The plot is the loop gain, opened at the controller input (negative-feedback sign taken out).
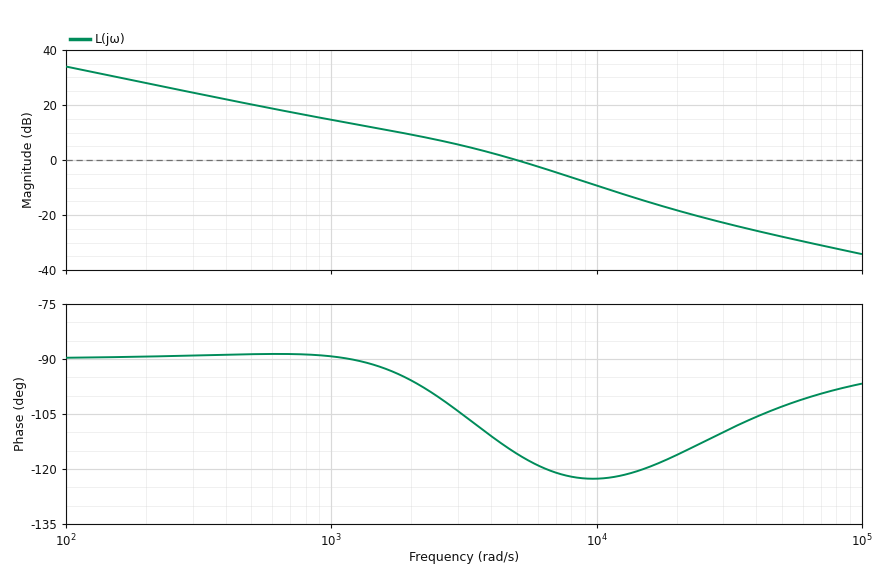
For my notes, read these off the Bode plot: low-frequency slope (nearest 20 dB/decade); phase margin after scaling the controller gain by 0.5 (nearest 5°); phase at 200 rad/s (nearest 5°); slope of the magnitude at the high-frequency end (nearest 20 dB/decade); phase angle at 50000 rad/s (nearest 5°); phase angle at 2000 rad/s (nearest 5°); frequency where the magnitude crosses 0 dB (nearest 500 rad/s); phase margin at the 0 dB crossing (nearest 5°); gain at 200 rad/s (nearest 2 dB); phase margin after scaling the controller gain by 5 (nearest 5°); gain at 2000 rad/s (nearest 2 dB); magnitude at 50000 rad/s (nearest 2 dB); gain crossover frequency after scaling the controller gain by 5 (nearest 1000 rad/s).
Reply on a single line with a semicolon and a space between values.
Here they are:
-20 dB/decade; 75°; -90°; -20 dB/decade; -105°; -95°; 5000 rad/s; 65°; 28 dB; 60°; 10 dB; -28 dB; 14000 rad/s
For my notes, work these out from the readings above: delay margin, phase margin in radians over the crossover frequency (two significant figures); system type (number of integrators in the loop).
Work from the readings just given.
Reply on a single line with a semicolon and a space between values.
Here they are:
0.00023 s; 1
